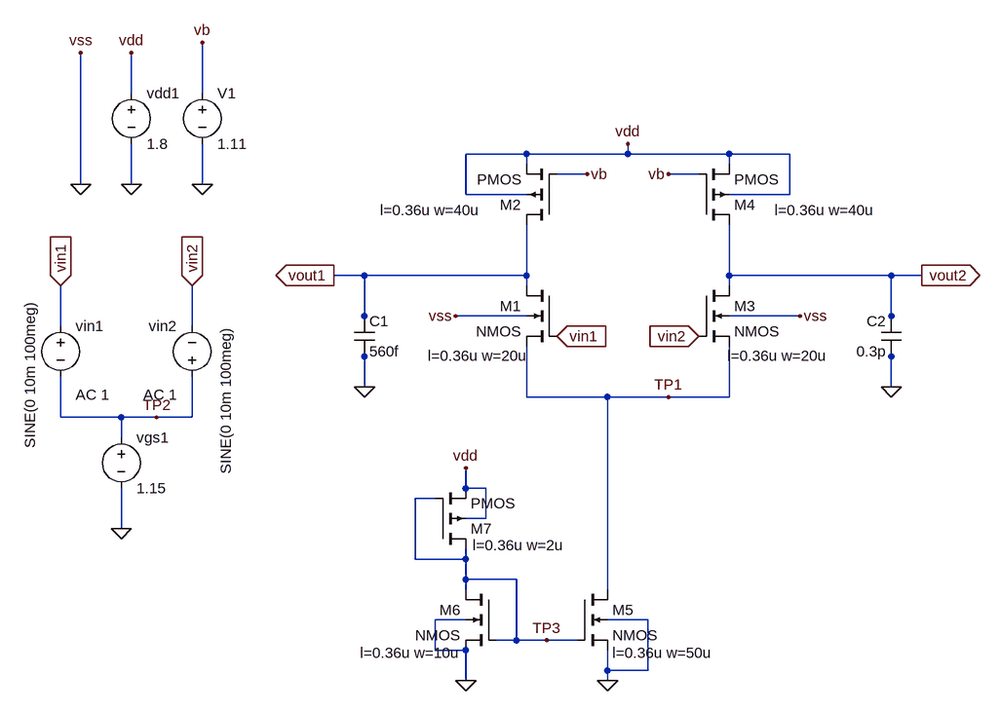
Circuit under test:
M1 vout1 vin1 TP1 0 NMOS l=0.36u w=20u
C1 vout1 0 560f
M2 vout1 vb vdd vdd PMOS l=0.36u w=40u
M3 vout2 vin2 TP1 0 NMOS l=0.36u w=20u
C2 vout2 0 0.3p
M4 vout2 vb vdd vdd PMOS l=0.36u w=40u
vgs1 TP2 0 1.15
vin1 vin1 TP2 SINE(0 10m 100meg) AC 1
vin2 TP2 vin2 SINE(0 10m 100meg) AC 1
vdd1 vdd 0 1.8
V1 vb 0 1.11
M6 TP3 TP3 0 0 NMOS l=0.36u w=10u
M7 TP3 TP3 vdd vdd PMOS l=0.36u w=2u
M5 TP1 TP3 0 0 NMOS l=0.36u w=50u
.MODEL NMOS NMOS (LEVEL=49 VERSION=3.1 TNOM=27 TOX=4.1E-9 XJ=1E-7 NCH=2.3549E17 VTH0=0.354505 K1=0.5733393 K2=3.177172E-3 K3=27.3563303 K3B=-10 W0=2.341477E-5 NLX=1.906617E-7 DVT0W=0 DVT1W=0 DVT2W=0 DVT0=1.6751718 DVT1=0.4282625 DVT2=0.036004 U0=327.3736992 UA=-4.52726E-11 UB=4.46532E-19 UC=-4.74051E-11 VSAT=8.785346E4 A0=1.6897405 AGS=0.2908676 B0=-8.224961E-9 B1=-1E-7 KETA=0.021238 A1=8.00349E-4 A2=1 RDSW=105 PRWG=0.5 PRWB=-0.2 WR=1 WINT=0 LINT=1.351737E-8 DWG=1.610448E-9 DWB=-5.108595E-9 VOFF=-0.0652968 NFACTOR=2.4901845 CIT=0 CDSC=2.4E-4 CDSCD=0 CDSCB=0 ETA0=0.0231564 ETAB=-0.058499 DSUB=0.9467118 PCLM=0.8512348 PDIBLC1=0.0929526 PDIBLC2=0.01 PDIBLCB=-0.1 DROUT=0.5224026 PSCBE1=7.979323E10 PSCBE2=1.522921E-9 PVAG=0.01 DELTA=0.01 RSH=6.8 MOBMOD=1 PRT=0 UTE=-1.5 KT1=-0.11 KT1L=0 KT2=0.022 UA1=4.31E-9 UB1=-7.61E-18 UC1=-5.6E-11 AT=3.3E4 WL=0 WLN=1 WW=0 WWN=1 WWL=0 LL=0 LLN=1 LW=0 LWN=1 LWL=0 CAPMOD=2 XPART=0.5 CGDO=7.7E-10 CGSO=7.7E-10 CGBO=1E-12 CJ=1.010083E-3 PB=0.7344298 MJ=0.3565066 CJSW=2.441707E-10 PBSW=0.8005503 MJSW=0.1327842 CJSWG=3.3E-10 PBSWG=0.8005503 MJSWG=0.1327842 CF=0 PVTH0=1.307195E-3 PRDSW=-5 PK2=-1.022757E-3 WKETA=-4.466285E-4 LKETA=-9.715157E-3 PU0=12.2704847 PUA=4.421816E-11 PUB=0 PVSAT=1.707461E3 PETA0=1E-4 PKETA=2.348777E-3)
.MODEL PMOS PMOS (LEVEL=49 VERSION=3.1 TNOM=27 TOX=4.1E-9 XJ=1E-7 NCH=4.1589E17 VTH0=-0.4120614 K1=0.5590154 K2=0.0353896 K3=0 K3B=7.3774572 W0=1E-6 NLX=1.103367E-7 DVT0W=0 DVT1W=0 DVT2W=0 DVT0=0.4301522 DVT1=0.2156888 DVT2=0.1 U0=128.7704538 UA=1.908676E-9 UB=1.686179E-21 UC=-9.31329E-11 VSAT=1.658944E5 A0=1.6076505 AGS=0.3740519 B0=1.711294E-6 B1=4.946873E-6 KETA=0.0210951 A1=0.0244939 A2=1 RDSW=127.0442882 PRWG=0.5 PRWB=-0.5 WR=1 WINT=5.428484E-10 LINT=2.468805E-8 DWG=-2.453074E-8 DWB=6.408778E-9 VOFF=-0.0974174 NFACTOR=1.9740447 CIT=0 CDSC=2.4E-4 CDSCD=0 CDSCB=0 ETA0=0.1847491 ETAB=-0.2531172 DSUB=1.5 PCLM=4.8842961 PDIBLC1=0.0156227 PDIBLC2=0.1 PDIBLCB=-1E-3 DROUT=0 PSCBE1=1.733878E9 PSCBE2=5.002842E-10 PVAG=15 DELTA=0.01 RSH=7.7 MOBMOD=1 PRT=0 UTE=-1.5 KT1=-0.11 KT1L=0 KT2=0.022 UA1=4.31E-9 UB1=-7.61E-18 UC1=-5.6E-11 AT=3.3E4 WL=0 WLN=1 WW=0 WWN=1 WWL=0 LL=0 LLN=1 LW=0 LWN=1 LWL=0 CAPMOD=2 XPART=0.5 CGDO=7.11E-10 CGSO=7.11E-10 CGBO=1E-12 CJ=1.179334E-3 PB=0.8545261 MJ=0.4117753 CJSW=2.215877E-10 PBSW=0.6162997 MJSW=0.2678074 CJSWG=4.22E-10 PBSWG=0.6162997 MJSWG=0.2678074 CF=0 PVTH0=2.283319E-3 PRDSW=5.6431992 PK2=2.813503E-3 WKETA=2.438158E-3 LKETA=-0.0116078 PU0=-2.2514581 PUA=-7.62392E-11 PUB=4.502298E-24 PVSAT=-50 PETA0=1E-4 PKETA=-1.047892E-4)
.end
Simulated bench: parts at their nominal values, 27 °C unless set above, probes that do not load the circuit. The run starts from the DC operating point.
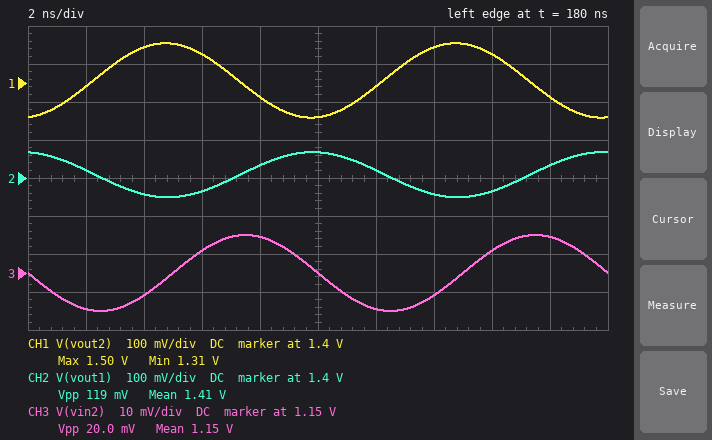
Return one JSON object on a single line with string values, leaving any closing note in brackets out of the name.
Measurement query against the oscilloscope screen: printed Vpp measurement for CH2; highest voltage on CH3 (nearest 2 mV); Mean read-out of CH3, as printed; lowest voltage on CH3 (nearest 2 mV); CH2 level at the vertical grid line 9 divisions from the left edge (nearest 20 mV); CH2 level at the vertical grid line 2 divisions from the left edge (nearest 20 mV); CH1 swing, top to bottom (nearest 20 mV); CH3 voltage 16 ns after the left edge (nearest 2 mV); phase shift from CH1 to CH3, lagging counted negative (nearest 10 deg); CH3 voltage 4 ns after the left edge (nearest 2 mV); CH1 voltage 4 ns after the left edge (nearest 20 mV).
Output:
{"printed Vpp measurement for CH2": "119 mV", "highest voltage on CH3": "1.160 V", "Mean read-out of CH3, as printed": "1.15 V", "lowest voltage on CH3": "1.140 V", "CH2 level at the vertical grid line 9 divisions from the left edge": "1.44 V", "CH2 level at the vertical grid line 2 divisions from the left edge": "1.36 V", "CH1 swing, top to bottom": "200 mV", "CH3 voltage 16 ns after the left edge": "1.156 V", "phase shift from CH1 to CH3, lagging counted negative": "-100 deg", "CH3 voltage 4 ns after the left edge": "1.144 V", "CH1 voltage 4 ns after the left edge": "1.50 V"}
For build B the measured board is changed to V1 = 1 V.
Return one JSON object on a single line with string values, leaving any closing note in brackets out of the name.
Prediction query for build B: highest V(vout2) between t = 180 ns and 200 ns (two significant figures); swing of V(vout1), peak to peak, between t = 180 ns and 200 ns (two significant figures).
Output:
{"highest V(vout2) between t = 180 ns and 200 ns": "1.7 V", "swing of V(vout1), peak to peak, between t = 180 ns and 200 ns": "24 mV"}
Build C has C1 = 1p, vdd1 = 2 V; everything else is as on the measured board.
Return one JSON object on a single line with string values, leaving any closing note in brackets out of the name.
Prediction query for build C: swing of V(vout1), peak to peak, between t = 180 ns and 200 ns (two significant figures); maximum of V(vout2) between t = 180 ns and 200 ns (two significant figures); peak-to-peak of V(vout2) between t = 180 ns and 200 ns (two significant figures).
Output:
{"swing of V(vout1), peak to peak, between t = 180 ns and 200 ns": "22 mV", "maximum of V(vout2) between t = 180 ns and 200 ns": "1.9 V", "peak-to-peak of V(vout2) between t = 180 ns and 200 ns": "23 mV"}
